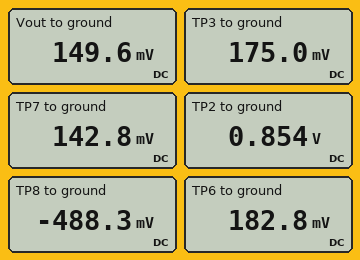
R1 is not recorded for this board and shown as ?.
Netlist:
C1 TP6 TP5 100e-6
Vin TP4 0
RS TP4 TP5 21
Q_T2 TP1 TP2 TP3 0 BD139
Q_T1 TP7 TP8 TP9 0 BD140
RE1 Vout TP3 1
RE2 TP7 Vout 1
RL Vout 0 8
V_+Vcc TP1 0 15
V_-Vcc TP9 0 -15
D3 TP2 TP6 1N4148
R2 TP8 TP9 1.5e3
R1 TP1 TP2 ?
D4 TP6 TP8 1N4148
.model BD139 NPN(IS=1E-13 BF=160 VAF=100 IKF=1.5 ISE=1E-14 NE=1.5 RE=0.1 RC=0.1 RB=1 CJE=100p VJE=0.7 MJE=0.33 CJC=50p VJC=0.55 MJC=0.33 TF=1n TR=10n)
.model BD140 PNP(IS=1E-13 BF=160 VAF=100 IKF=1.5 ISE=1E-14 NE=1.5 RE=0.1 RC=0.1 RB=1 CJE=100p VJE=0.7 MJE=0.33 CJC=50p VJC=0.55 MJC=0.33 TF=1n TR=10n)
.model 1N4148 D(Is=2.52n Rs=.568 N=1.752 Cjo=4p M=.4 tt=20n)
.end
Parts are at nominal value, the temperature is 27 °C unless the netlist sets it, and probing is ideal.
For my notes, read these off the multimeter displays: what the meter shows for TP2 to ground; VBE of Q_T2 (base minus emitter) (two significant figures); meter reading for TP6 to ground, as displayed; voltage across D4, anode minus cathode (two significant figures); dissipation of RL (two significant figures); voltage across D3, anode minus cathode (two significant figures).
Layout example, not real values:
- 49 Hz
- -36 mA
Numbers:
- 0.854 V
- 680 mV
- 182.8 mV
- 670 mV
- 2.8 mW
- 670 mV
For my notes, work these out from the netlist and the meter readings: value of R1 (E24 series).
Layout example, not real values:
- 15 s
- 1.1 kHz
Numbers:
- 2.2 kΩ
